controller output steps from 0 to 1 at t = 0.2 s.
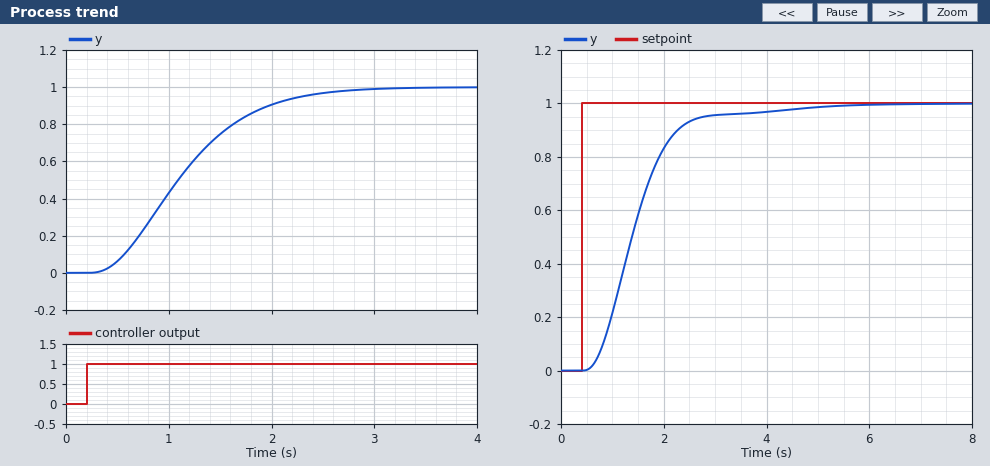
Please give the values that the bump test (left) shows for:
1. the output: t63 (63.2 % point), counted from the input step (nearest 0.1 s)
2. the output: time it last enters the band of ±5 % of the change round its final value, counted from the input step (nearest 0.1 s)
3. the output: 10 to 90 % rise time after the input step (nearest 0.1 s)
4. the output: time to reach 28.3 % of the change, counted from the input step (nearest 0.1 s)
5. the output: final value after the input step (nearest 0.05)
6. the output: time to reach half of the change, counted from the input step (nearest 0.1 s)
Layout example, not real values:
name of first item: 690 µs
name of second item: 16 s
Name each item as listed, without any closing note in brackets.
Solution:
the output: t63 (63.2 % point), counted from the input step: 1.1 s
the output: time it last enters the band of ±5 % of the change round its final value, counted from the input step: 2.1 s
the output: 10 to 90 % rise time after the input step: 1.4 s
the output: time to reach 28.3 % of the change, counted from the input step: 0.6 s
the output: final value after the input step: 1.00
the output: time to reach half of the change, counted from the input step: 0.9 s
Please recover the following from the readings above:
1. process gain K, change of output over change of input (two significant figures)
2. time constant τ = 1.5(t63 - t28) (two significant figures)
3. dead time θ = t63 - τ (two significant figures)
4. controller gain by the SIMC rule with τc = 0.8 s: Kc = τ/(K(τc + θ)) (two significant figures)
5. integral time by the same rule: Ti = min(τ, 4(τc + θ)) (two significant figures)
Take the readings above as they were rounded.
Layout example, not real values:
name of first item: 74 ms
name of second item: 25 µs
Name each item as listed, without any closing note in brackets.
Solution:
process gain K, change of output over change of input: 1.0
time constant τ = 1.5(t63 - t28): 0.75 s
dead time θ = t63 - τ: 0.35 s
controller gain by the SIMC rule with τc = 0.8 s: Kc = τ/(K(τc + θ)): 0.65
integral time by the same rule: Ti = min(τ, 4(τc + θ)): 0.75 s
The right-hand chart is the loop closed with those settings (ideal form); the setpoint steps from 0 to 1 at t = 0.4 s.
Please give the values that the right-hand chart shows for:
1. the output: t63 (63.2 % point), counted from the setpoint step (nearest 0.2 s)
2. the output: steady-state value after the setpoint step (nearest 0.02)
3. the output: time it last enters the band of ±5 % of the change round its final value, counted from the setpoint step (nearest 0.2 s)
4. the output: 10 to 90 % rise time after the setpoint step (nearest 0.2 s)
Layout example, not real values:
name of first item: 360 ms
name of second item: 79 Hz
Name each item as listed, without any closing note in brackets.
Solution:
the output: t63 (63.2 % point), counted from the setpoint step: 1.2 s
the output: steady-state value after the setpoint step: 1.00
the output: time it last enters the band of ±5 % of the change round its final value, counted from the setpoint step: 2.4 s
the output: 10 to 90 % rise time after the setpoint step: 1.4 s
